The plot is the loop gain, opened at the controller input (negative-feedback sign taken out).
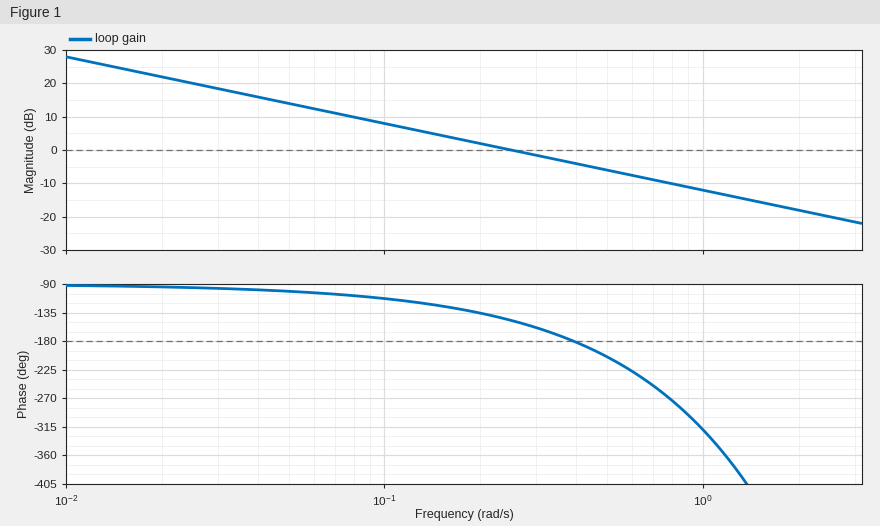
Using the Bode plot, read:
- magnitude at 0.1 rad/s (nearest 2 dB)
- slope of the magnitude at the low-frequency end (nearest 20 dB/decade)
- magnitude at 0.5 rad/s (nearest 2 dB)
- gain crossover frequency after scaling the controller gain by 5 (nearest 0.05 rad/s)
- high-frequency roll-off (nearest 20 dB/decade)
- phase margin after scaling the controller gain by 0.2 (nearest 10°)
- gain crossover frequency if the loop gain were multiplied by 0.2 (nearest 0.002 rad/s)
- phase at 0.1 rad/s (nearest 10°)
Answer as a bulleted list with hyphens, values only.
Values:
- 8 dB
- -20 dB/decade
- -6 dB
- 1.25 rad/s
- -20 dB/decade
- 80°
- 0.050 rad/s
- -110°
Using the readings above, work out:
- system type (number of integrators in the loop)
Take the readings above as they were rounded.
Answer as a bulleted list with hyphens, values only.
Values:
- 1
